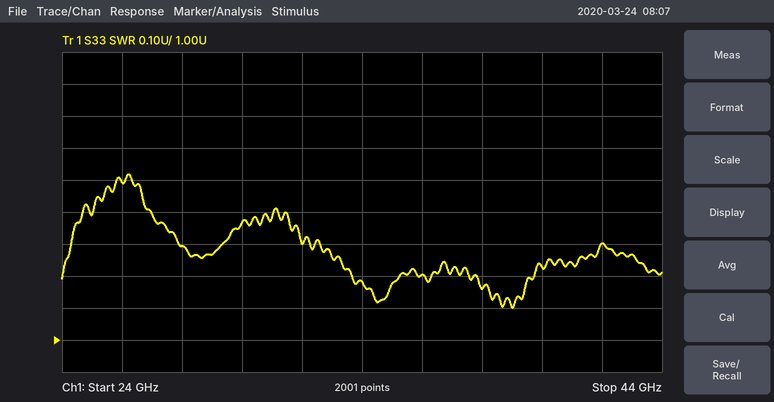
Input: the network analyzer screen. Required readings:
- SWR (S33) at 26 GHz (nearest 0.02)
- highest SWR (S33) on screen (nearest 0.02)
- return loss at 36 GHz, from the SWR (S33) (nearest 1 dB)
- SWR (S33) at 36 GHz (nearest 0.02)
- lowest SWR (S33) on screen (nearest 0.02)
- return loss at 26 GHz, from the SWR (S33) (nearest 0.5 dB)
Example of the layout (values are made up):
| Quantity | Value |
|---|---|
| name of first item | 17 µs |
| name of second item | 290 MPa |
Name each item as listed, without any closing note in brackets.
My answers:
| Quantity | Value |
|---|---|
| SWR (S33) at 26 GHz | 1.50 |
| highest SWR (S33) on screen | 1.52 |
| return loss at 36 GHz, from the SWR (S33) | 21 dB |
| SWR (S33) at 36 GHz | 1.20 |
| lowest SWR (S33) on screen | 1.10 |
| return loss at 26 GHz, from the SWR (S33) | 14.0 dB |
